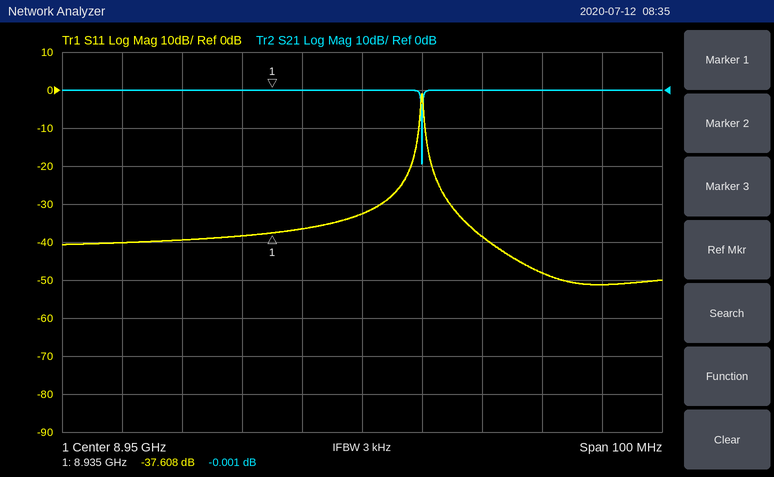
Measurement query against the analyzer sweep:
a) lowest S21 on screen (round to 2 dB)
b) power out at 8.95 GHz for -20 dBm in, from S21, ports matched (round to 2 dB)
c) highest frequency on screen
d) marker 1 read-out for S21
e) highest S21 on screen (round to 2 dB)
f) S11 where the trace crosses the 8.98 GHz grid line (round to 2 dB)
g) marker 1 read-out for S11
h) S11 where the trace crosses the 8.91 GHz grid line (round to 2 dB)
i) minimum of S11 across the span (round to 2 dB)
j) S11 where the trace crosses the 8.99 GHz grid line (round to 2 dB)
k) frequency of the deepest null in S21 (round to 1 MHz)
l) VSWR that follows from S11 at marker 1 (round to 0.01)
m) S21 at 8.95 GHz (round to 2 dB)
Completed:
-20 dB
-20 dBm
9 GHz
-0.001 dB
0 dB
-48 dB
-37.608 dB
-40 dB
-52 dB
-52 dB
8.960 GHz
1.03
0 dB
